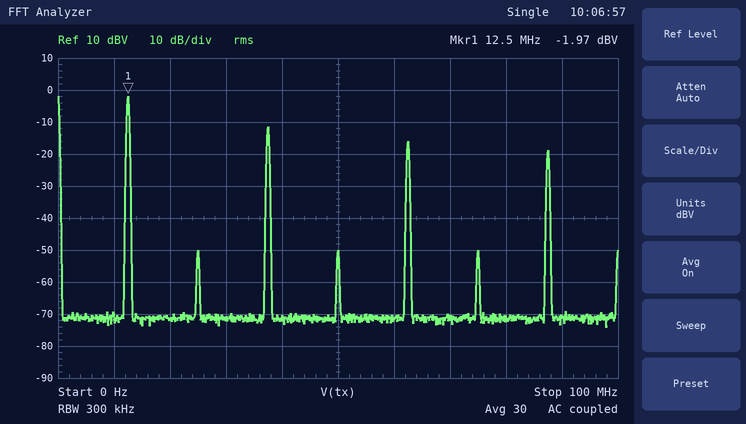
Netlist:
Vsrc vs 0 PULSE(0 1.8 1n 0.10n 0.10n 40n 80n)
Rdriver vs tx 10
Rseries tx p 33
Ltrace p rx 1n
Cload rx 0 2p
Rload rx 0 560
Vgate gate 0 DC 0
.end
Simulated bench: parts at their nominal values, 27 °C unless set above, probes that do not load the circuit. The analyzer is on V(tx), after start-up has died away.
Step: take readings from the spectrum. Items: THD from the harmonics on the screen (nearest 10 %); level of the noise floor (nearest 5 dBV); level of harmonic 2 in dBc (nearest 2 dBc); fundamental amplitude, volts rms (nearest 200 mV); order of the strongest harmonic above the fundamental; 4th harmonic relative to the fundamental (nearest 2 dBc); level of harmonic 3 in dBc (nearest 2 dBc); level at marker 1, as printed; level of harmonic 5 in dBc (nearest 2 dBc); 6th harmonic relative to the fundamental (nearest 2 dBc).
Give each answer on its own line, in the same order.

40 %
-70 dBV
-48 dBc
800 mV
3
-48 dBc
-10 dBc
-1.97 dBV
-14 dBc
-48 dBc
